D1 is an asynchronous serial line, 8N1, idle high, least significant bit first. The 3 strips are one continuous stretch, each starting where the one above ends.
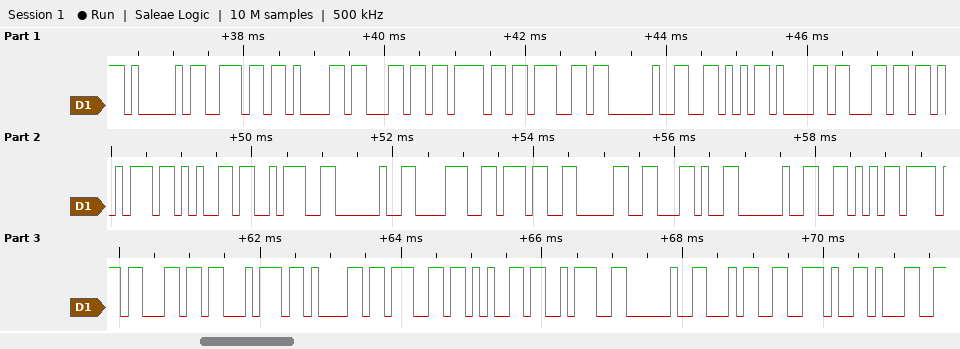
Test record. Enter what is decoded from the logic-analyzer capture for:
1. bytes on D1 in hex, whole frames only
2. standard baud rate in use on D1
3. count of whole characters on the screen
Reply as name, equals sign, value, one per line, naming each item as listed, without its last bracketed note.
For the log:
bytes on D1 in hex, whole frames only = 41 6E 61 6C 6F 67 20 56 61 6C 75 65 3A 20 38 37 30 2C 20 56 6F 6C 74 61 67 65 3A 20 34 2E 31
standard baud rate in use on D1 = 9600 baud
count of whole characters on the screen = 31
